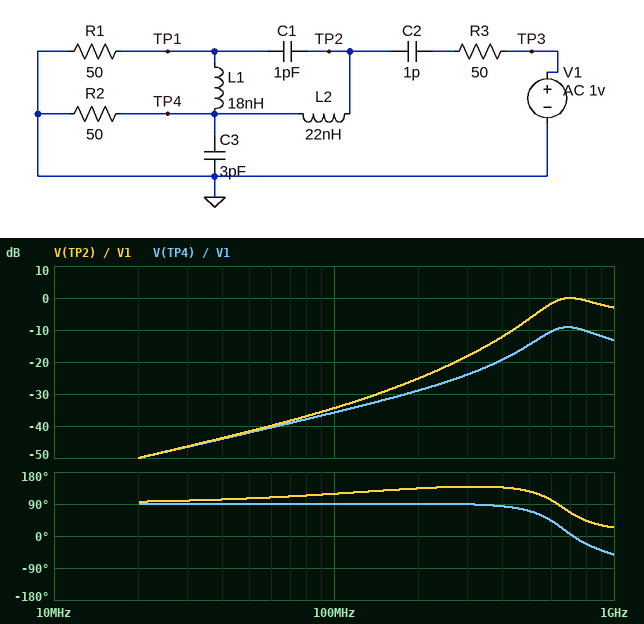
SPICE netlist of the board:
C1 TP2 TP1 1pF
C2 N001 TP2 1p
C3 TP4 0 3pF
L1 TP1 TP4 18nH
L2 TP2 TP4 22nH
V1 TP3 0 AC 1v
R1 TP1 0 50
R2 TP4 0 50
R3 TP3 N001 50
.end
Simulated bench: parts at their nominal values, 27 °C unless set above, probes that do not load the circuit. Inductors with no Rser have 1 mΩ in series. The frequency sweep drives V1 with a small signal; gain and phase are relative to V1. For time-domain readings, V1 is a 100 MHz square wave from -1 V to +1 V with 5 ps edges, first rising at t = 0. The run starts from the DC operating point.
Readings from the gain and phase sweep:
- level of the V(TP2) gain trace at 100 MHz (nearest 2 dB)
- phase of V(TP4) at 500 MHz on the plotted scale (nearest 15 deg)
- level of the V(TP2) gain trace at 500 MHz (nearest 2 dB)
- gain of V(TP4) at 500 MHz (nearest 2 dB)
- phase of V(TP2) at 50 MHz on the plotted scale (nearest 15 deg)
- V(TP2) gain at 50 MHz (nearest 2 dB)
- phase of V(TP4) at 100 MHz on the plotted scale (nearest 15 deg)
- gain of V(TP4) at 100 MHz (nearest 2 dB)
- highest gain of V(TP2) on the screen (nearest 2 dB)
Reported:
-34 dB
75 deg
-6 dB
-14 dB
105 deg
-42 dB
90 deg
-36 dB
0 dB
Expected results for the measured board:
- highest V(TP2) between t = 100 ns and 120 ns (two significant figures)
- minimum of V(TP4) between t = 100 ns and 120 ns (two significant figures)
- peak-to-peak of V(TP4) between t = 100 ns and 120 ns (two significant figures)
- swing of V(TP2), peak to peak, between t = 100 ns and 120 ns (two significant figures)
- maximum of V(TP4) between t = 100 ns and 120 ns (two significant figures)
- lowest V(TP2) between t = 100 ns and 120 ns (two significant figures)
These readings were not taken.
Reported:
990 mV
-230 mV
470 mV
2.0 V
230 mV
-990 mV
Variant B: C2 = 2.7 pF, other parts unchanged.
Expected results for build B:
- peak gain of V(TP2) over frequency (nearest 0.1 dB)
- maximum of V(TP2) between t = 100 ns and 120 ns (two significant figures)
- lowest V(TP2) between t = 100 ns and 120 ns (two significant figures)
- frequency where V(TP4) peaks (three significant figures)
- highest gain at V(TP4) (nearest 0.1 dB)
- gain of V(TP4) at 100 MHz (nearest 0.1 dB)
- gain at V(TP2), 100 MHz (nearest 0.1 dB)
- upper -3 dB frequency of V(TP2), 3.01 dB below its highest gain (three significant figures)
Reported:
1.1 dB
1.1 V
-1.1 V
529 MHz
-7.3 dB
-27.1 dB
-25.7 dB
1.01 GHz
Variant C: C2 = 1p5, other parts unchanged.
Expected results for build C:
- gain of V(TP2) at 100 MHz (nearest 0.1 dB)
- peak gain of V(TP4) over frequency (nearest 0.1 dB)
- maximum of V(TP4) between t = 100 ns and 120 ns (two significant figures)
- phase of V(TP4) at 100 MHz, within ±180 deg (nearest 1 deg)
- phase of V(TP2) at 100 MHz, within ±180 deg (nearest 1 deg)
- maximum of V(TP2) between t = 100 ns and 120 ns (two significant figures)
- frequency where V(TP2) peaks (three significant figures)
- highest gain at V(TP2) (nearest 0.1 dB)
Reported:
-30.9 dB
-7.9 dB
290 mV
90 deg
117 deg
1.0 V
635 MHz
1.0 dB
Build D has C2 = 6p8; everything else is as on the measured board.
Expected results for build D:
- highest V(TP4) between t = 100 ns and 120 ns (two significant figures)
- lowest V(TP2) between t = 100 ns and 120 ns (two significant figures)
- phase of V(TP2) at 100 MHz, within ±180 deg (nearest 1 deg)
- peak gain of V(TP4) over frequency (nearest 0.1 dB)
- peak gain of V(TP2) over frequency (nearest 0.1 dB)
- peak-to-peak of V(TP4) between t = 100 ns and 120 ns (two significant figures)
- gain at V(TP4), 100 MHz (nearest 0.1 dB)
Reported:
510 mV
-1.3 V
102 deg
-7.9 dB
-0.2 dB
1.0 V
-19.1 dB
